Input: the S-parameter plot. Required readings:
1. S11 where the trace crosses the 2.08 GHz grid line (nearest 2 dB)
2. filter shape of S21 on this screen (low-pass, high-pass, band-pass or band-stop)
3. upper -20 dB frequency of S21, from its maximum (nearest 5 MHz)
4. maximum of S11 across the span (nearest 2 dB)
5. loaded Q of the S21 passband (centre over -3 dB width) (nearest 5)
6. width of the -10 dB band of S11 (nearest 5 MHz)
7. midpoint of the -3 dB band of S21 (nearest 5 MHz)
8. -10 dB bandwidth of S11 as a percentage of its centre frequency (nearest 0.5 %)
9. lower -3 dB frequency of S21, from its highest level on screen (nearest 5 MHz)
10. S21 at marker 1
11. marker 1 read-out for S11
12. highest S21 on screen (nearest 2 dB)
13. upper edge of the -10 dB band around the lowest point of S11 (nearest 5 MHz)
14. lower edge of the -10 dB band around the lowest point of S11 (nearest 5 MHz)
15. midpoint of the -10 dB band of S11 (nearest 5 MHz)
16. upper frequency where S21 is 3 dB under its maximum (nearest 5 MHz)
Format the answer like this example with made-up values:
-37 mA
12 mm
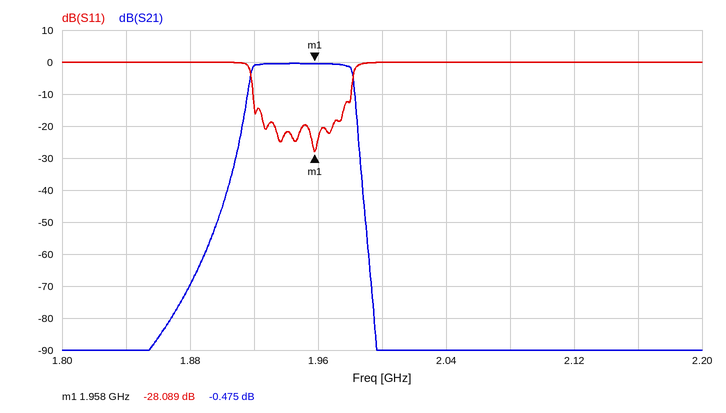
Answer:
0 dB
band-pass
1.985 GHz
0 dB
30
60 MHz
1.950 GHz
3.0 %
1.920 GHz
-0.475 dB
-28.089 dB
0 dB
1.980 GHz
1.920 GHz
1.950 GHz
1.980 GHz
